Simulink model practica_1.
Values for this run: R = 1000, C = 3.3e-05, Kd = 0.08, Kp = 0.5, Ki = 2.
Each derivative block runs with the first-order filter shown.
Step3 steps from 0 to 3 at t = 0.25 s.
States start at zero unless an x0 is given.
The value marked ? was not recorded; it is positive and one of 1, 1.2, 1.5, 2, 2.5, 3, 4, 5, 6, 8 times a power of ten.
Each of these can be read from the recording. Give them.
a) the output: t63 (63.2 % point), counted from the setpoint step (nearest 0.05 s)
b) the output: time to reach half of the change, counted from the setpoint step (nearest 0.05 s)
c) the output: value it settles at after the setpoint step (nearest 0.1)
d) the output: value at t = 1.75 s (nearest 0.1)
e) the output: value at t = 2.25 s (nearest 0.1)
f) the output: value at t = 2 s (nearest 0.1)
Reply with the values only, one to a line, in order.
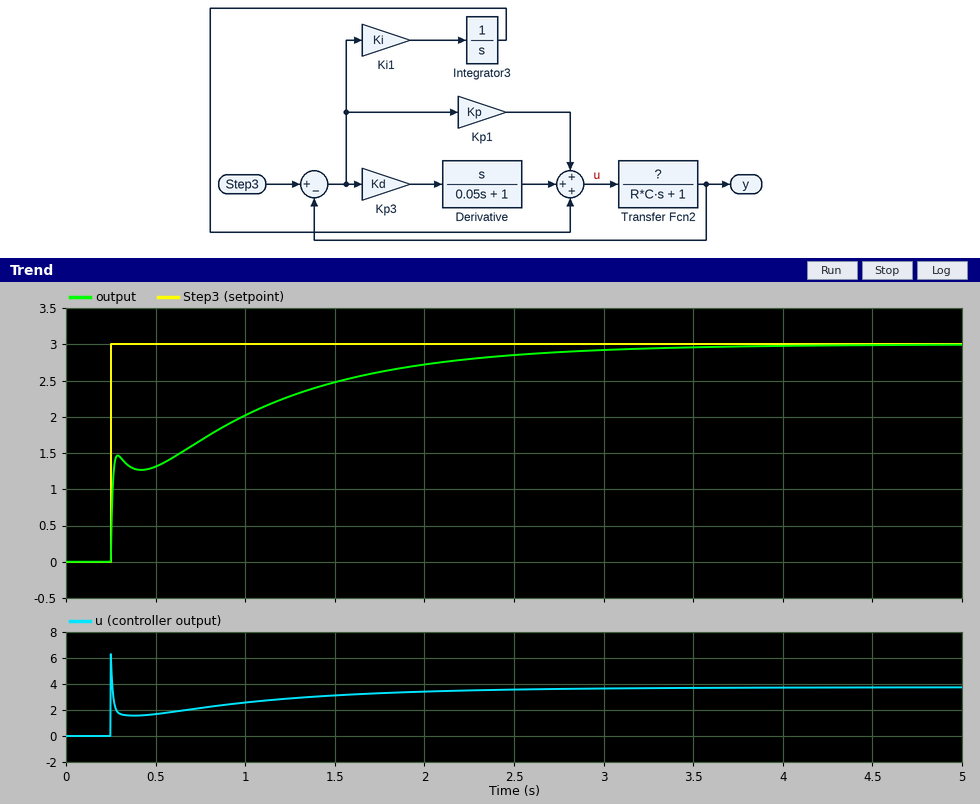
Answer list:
0.65 s
0.40 s
3.0
2.6
2.8
2.7
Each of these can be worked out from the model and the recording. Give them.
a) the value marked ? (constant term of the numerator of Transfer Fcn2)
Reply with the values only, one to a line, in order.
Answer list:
0.8
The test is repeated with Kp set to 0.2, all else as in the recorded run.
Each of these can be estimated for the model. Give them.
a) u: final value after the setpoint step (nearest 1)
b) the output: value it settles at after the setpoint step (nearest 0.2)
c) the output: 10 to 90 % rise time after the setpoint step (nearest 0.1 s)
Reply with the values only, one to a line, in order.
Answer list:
4
3.0
1.5 s
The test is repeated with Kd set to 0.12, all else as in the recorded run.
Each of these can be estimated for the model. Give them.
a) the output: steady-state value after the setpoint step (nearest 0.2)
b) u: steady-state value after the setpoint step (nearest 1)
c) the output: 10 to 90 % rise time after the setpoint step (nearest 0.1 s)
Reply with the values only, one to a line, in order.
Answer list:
3.0
4
1.7 s
